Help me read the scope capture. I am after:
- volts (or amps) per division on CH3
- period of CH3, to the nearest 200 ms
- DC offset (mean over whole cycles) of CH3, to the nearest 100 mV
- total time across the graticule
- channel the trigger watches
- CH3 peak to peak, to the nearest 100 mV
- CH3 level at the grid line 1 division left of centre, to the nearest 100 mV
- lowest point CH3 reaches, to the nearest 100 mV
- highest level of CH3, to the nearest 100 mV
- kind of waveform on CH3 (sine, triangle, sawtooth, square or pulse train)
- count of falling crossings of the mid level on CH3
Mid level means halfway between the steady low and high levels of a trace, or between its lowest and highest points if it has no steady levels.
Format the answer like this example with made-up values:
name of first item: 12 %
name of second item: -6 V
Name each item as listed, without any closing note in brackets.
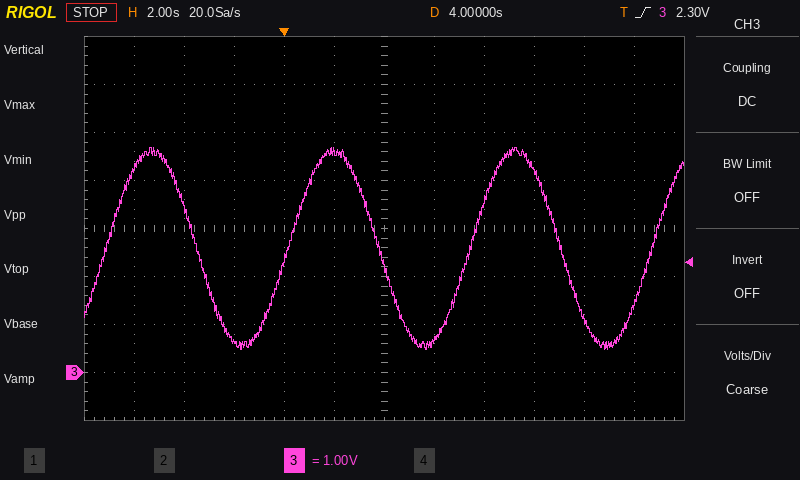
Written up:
volts (or amps) per division on CH3: 1 V
period of CH3, to the nearest 200 ms: 7.2 s
DC offset (mean over whole cycles) of CH3, to the nearest 100 mV: 2.6 V
total time across the graticule: 24 s
channel the trigger watches: CH3
CH3 peak to peak, to the nearest 100 mV: 4.2 V
CH3 level at the grid line 1 division left of centre, to the nearest 100 mV: 4.6 V
lowest point CH3 reaches, to the nearest 100 mV: 500 mV
highest level of CH3, to the nearest 100 mV: 4.7 V
kind of waveform on CH3: sine
count of falling crossings of the mid level on CH3: 3
